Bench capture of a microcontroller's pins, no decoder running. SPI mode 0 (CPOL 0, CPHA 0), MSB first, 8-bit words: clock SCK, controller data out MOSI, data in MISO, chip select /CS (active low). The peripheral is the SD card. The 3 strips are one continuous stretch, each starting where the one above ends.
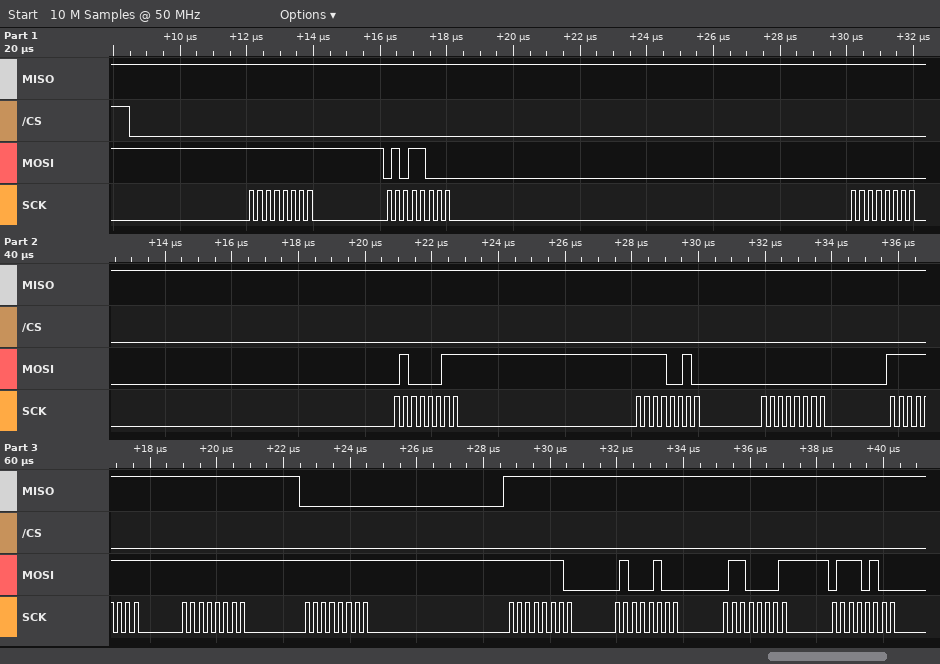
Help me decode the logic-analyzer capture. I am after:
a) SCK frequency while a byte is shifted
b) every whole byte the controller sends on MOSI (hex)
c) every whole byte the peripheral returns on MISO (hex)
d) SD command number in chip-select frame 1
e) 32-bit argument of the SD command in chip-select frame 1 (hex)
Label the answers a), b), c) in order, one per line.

a) 4 MHz
b) 0xFF 0x58 0x00 0x43 0xF2 0x00 0xFF 0xFF 0xFF 0xFE 0x44 0x61 0x74
c) 0xFF 0xFF 0xFF 0xFF 0xFF 0xFF 0xFF 0xFF 0x00 0xFF 0xFF 0xFF 0xFF
d) CMD24
e) 0x0043F200
